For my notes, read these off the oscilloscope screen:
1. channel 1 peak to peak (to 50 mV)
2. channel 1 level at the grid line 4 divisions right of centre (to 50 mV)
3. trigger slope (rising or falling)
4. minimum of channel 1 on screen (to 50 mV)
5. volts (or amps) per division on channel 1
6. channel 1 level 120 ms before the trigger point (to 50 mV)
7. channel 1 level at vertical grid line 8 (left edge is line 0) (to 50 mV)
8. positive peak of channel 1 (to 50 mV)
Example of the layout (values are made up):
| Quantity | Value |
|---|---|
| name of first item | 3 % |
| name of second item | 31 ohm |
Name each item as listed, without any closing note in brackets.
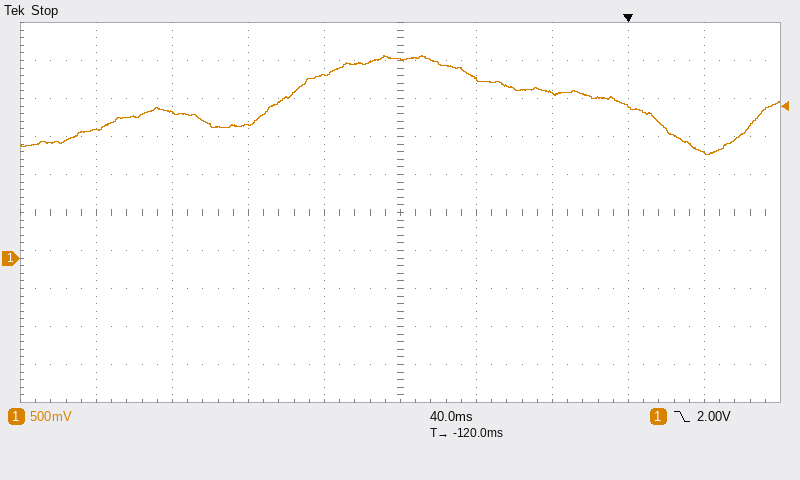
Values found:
| Quantity | Value |
|---|---|
| channel 1 peak to peak | 1.30 V |
| channel 1 level at the grid line 4 divisions right of centre | 1.40 V |
| trigger slope | falling |
| minimum of channel 1 on screen | 1.35 V |
| volts (or amps) per division on channel 1 | 500 mV |
| channel 1 level 120 ms before the trigger point | 2.60 V |
| channel 1 level at vertical grid line 8 (left edge is line 0) | 2.00 V |
| positive peak of channel 1 | 2.65 V |
